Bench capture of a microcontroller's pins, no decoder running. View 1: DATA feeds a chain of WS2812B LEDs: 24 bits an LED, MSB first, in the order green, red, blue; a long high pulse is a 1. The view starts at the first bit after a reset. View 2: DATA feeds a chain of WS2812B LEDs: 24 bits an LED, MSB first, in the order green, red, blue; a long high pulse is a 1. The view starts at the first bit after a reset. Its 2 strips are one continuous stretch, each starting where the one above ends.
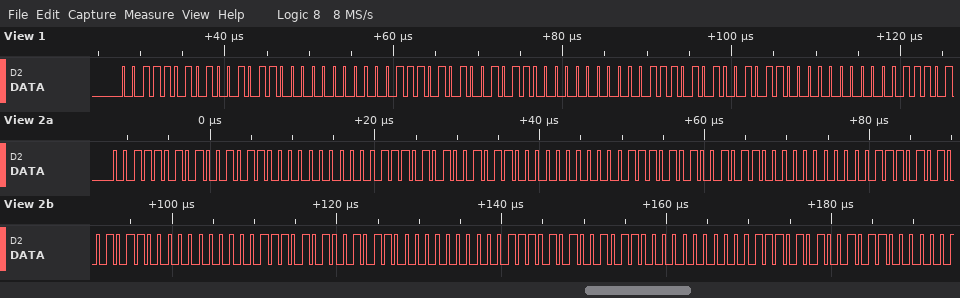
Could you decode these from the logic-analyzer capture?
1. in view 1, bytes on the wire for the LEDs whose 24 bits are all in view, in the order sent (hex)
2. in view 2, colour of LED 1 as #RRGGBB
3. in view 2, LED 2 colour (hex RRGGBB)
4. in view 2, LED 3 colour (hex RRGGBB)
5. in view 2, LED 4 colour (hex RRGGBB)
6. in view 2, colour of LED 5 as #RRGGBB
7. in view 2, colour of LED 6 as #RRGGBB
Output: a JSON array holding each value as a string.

["3A 96 00 3A 96 00 3A 96 00", "#963A00", "#963A00", "#963A00", "#963A00", "#963A00", "#963A00"]
